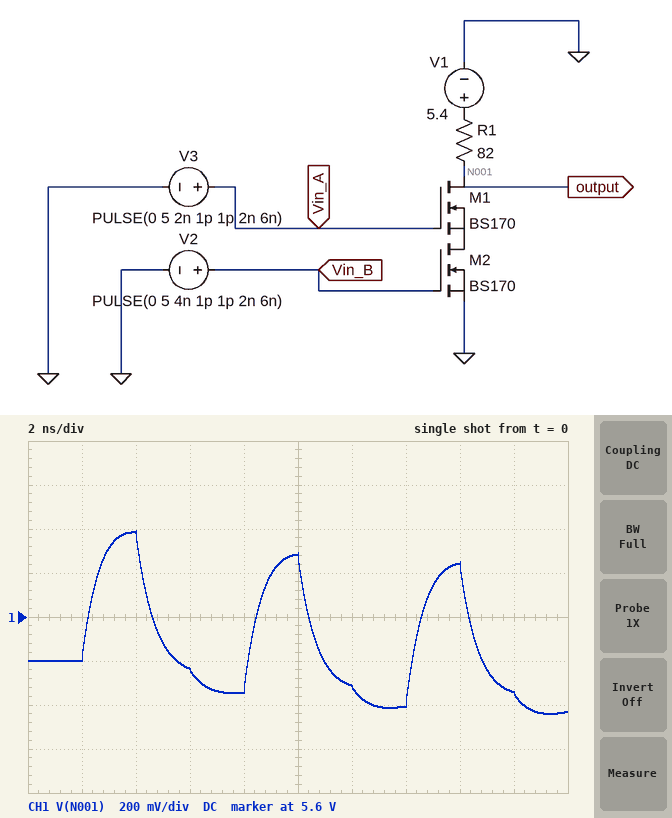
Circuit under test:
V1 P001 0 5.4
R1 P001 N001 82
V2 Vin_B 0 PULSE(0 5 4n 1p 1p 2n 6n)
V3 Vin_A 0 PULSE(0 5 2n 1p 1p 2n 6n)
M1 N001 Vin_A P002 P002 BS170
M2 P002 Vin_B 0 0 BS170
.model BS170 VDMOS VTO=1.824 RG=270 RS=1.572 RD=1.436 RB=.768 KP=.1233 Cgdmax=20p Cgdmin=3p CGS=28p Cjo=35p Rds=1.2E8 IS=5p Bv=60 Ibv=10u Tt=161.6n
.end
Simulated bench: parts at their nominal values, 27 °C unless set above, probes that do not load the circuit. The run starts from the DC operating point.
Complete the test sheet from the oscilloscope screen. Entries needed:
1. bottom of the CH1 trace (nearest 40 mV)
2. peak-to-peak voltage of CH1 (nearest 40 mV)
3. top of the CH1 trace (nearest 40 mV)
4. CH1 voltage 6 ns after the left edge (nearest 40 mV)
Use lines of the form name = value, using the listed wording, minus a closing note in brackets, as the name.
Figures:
bottom of the CH1 trace = 5.16 V
peak-to-peak voltage of CH1 = 840 mV
top of the CH1 trace = 6.00 V
CH1 voltage 6 ns after the left edge = 5.36 V
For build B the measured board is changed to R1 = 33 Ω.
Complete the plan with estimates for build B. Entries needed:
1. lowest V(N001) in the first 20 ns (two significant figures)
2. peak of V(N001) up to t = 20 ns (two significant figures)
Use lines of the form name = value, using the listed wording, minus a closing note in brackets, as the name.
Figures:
lowest V(N001) in the first 20 ns = 5.3 V
peak of V(N001) up to t = 20 ns = 5.7 V
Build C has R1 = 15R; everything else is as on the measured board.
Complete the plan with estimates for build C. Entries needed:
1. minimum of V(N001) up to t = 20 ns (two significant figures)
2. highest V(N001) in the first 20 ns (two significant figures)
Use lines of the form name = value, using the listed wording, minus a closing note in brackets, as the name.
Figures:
minimum of V(N001) up to t = 20 ns = 5.3 V
highest V(N001) in the first 20 ns = 5.5 V
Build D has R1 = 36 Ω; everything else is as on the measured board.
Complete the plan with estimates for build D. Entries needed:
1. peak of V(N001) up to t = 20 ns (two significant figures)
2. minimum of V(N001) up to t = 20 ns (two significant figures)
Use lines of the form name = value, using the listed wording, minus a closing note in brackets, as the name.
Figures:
peak of V(N001) up to t = 20 ns = 5.7 V
minimum of V(N001) up to t = 20 ns = 5.3 V
